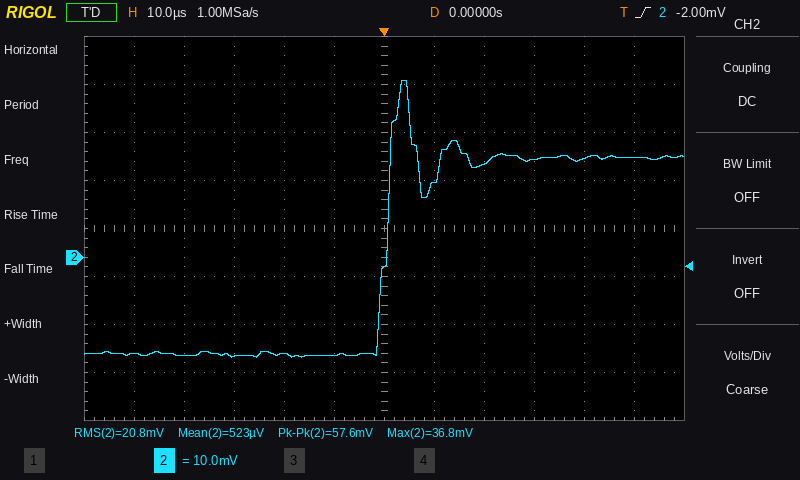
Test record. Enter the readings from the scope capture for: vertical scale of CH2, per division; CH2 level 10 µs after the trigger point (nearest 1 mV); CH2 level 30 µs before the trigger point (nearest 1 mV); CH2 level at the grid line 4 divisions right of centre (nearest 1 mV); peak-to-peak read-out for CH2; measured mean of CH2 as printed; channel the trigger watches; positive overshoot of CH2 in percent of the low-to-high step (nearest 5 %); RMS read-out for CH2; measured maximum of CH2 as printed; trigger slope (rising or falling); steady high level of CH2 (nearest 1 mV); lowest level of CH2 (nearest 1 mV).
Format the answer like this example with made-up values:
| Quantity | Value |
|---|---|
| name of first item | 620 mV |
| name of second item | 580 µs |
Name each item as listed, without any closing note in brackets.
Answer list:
| Quantity | Value |
|---|---|
| vertical scale of CH2, per division | 10 mV |
| CH2 level 10 µs after the trigger point | 16 mV |
| CH2 level 30 µs before the trigger point | -21 mV |
| CH2 level at the grid line 4 divisions right of centre | 21 mV |
| peak-to-peak read-out for CH2 | 57.6 mV |
| measured mean of CH2 as printed | 523 µV |
| channel the trigger watches | CH2 |
| positive overshoot of CH2 in percent of the low-to-high step | 40 % |
| RMS read-out for CH2 | 20.8 mV |
| measured maximum of CH2 as printed | 36.8 mV |
| trigger slope | rising |
| steady high level of CH2 | 21 mV |
| lowest level of CH2 | -21 mV |
